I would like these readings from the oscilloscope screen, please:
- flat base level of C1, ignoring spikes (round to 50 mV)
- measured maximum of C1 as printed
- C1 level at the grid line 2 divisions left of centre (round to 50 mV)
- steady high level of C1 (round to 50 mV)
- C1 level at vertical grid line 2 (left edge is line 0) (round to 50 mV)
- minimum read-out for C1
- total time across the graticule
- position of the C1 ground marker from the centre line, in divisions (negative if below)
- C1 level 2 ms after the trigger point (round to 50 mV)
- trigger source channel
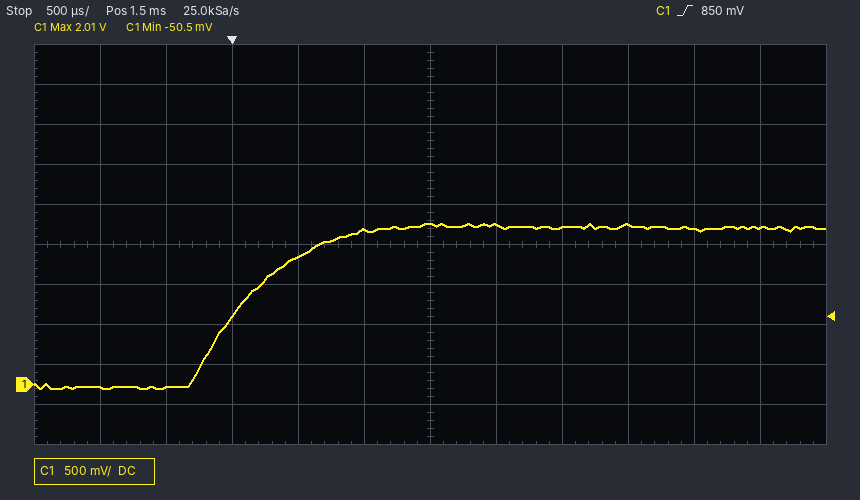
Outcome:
0 mV
2.01 V
1.60 V
2.00 V
-50 mV
-50.5 mV
6 ms
-3.5 div
2.00 V
C1
